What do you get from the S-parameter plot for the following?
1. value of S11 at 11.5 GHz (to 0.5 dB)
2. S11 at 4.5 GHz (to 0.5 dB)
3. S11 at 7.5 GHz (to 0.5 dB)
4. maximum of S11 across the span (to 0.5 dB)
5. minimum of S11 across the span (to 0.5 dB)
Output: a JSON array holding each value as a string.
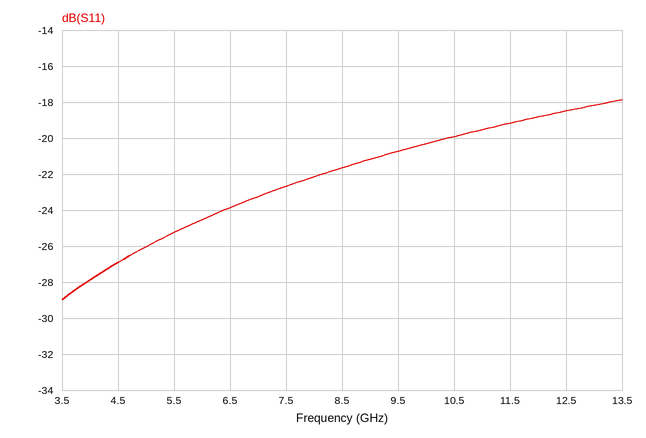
["-19.0 dB", "-27.0 dB", "-22.5 dB", "-18.0 dB", "-29.0 dB"]
